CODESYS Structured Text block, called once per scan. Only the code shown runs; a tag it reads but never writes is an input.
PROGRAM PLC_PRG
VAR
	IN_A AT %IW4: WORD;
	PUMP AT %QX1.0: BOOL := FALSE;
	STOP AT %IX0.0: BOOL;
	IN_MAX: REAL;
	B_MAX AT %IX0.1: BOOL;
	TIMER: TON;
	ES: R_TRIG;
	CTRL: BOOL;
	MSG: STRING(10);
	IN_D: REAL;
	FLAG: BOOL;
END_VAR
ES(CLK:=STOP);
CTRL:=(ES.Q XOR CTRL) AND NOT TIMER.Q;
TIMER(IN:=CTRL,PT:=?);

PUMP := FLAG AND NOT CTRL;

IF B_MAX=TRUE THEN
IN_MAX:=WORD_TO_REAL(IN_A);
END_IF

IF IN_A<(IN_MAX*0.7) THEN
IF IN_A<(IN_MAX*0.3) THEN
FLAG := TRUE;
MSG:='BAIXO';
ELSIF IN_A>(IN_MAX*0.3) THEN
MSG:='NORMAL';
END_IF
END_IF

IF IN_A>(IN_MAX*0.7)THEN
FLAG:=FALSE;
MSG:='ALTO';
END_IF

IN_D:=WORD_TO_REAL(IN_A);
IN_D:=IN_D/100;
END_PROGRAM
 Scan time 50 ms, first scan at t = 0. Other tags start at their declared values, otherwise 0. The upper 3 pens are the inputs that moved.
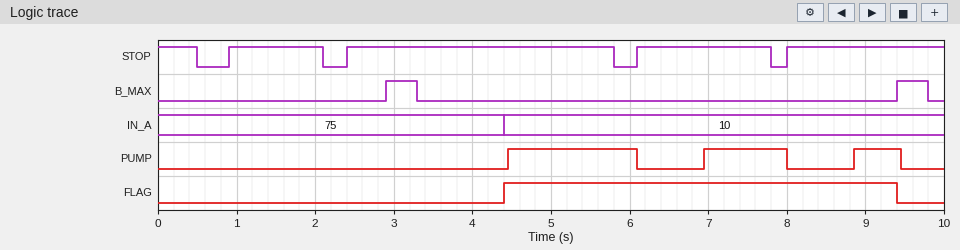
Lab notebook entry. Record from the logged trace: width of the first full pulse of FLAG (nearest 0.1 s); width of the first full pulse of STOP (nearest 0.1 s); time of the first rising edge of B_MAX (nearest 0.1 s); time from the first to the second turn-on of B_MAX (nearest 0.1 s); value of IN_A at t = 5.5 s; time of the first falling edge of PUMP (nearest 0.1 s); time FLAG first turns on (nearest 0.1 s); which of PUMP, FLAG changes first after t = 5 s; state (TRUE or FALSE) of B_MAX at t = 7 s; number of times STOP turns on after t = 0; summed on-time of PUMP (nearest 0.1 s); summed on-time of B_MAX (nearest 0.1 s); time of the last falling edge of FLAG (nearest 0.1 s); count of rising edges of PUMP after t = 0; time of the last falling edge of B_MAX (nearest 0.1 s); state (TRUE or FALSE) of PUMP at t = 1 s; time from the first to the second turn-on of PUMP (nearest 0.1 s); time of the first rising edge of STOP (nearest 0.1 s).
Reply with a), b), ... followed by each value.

a) 5.0 s
b) 1.2 s
c) 2.9 s
d) 6.5 s
e) 10
f) 6.1 s
g) 4.4 s
h) PUMP
i) FALSE
j) 4
k) 3.3 s
l) 0.8 s
m) 9.4 s
n) 3
o) 9.8 s
p) FALSE
q) 2.5 s
r) 0.9 s
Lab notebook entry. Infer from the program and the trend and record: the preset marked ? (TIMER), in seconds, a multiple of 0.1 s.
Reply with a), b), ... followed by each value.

a) 0.8 s
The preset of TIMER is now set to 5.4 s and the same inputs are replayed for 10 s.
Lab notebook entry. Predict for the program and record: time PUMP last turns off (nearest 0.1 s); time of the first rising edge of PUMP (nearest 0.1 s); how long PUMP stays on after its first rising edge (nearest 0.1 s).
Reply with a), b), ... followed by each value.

a) 8.0 s
b) 6.1 s
c) 1.9 s
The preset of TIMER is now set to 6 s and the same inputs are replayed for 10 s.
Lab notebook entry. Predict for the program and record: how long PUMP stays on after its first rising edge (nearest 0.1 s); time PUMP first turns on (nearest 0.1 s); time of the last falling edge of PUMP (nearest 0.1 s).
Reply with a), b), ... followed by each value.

a) 1.9 s
b) 6.1 s
c) 8.0 s
